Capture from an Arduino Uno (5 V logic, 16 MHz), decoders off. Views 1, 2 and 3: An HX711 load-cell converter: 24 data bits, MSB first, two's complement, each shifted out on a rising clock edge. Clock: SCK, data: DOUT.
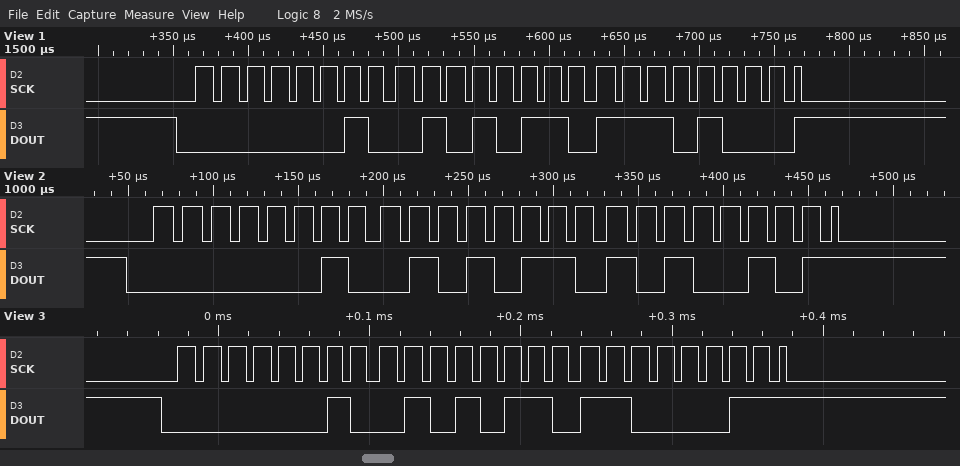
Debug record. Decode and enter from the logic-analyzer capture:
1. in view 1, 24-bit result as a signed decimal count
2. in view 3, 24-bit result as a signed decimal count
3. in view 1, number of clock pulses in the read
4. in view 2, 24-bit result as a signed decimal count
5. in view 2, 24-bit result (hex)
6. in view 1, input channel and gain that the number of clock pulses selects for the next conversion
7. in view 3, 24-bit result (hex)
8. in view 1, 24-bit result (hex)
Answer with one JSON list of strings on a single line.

["153320", "153283", "25", "153253", "0x0256A5", "channel A, gain 128", "0x0256C3", "0x0256E8"]
